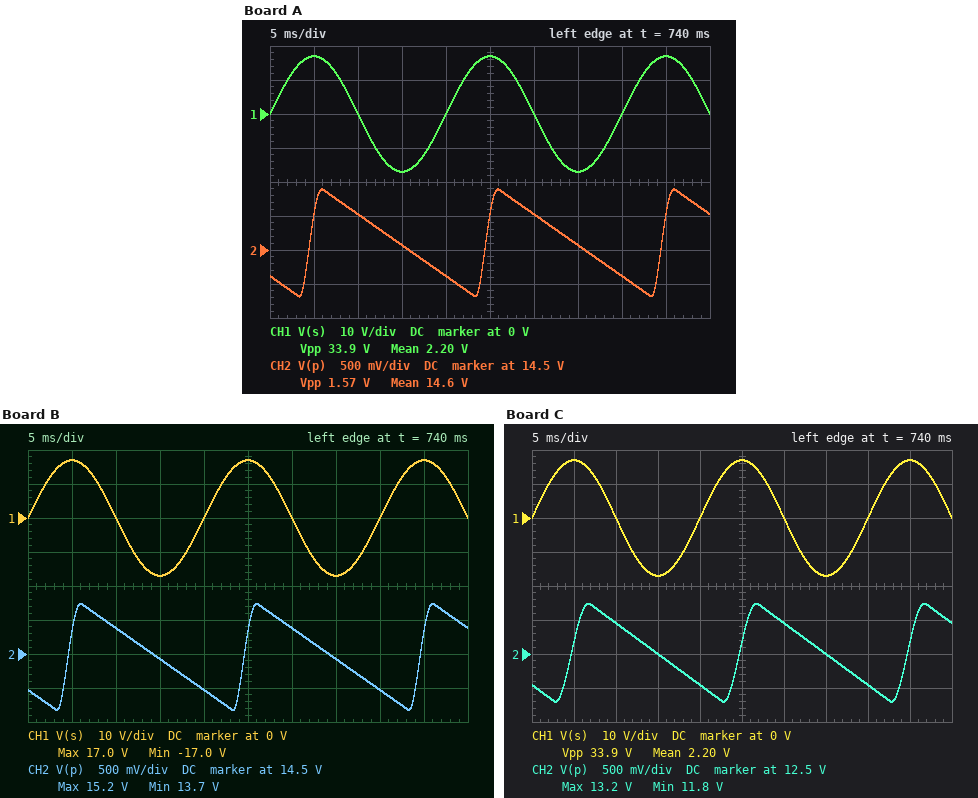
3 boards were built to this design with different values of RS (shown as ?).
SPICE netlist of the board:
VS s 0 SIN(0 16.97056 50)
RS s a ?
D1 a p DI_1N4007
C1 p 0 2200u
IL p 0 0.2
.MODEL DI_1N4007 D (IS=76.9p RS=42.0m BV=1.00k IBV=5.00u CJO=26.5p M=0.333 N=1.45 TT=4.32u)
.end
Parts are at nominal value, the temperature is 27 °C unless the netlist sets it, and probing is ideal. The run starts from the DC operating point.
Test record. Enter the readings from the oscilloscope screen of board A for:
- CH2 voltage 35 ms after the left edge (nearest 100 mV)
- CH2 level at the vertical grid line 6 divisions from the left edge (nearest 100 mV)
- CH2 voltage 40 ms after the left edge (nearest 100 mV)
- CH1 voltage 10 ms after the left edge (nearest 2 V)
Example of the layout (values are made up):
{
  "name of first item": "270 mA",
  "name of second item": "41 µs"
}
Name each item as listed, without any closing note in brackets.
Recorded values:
{
  "CH2 voltage 35 ms after the left edge": "14.6 V",
  "CH2 level at the vertical grid line 6 divisions from the left edge": "15.0 V",
  "CH2 voltage 40 ms after the left edge": "14.1 V",
  "CH1 voltage 10 ms after the left edge": "0 V"
}
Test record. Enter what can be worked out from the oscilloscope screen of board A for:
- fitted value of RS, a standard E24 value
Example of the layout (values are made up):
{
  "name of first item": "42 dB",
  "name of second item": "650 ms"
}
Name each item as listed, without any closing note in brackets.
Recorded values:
{
  "fitted value of RS, a standard E24 value": "0.51 Ω"
}
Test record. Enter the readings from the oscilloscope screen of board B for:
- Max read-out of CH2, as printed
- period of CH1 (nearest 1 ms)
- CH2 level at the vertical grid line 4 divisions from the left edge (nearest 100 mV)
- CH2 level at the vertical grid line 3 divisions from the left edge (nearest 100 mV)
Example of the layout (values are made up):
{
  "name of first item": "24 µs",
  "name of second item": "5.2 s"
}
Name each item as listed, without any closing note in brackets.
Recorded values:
{
  "Max read-out of CH2, as printed": "15.2 V",
  "period of CH1": "20 ms",
  "CH2 level at the vertical grid line 4 divisions from the left edge": "14.0 V",
  "CH2 level at the vertical grid line 3 divisions from the left edge": "14.4 V"
}
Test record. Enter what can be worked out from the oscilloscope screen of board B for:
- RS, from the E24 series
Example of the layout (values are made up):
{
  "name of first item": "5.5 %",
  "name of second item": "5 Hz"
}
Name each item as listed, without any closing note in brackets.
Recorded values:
{
  "RS, from the E24 series": "0.62 Ω"
}
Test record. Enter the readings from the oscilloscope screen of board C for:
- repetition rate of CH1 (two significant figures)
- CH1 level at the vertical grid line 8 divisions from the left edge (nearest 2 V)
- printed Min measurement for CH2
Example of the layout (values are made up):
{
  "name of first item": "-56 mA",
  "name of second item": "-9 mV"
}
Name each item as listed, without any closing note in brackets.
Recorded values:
{
  "repetition rate of CH1": "50 Hz",
  "CH1 level at the vertical grid line 8 divisions from the left edge": "0 V",
  "printed Min measurement for CH2": "11.8 V"
}
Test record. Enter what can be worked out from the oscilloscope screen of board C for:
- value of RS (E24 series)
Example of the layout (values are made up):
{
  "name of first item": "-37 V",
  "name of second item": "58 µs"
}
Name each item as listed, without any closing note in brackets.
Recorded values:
{
  "value of RS": "2.4 Ω"
}
